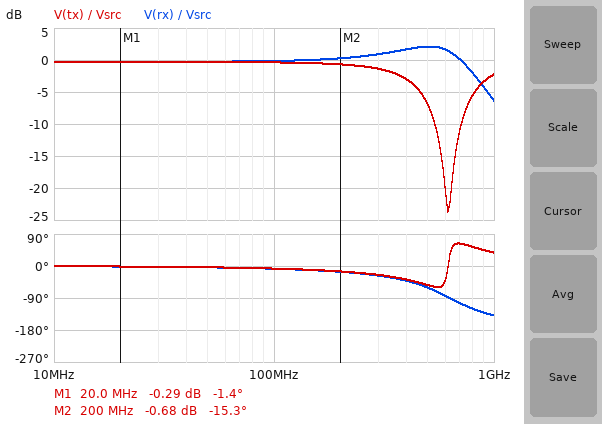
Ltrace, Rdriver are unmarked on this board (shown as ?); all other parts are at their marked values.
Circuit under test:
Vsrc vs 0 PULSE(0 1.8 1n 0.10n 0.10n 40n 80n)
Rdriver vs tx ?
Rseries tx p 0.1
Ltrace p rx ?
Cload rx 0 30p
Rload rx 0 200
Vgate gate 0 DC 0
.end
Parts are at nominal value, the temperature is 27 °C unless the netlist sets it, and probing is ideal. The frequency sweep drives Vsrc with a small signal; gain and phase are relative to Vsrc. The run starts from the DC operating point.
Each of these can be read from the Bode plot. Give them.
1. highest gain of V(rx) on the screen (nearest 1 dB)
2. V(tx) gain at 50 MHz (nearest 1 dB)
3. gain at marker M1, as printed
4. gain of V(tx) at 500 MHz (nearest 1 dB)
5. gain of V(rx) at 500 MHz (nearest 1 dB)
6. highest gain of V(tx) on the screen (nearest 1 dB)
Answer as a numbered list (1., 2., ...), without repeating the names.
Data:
1. 2 dB
2. 0 dB
3. -0.29 dB
4. -7 dB
5. 2 dB
6. 0 dB
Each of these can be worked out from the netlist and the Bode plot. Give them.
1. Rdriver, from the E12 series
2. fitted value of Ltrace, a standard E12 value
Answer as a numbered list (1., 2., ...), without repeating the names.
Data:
1. 6.8 Ω
2. 2.2 nH
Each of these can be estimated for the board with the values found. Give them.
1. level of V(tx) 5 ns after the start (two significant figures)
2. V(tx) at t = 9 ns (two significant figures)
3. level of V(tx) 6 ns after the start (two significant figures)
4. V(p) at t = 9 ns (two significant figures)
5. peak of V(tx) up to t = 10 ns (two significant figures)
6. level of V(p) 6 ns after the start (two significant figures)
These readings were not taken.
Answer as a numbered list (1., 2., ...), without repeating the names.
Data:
1. 1.7 V
2. 1.7 V
3. 1.7 V
4. 1.7 V
5. 1.9 V
6. 1.7 V
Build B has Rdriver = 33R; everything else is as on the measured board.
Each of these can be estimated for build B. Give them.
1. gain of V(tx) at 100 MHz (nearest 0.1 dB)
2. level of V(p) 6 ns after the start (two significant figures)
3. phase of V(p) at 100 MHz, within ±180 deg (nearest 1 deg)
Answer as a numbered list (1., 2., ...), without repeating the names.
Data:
1. -2.5 dB
2. 1.5 V
3. -29 deg
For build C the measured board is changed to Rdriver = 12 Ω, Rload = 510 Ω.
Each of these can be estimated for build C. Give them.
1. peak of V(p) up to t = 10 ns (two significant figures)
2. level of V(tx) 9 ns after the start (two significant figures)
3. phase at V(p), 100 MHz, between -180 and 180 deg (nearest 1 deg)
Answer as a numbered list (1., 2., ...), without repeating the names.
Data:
1. 1.8 V
2. 1.8 V
3. -13 deg
